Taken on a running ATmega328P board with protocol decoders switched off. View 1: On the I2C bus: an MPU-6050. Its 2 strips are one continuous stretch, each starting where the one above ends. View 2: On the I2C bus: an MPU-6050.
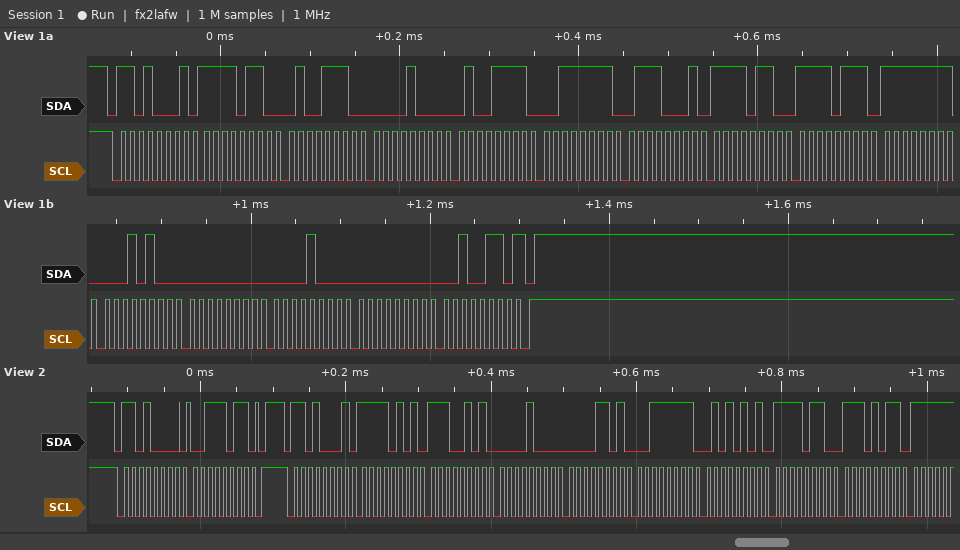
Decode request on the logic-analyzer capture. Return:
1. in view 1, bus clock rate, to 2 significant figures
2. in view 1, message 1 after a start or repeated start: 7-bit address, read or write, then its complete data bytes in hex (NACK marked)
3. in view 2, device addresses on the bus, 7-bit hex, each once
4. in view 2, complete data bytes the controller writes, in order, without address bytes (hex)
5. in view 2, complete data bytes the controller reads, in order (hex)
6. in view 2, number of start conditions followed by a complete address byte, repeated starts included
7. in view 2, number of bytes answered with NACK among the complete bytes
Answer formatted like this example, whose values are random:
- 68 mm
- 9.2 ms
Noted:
- 100 kHz
- 0x68 read: F6 4E 08 4F 3F 71 F6 F7 FF 14 00 08 00 26 NACK
- 0x68
- 3B
- F5 E5 08 0D 3F 55 F6 EB
- 2
- 0
